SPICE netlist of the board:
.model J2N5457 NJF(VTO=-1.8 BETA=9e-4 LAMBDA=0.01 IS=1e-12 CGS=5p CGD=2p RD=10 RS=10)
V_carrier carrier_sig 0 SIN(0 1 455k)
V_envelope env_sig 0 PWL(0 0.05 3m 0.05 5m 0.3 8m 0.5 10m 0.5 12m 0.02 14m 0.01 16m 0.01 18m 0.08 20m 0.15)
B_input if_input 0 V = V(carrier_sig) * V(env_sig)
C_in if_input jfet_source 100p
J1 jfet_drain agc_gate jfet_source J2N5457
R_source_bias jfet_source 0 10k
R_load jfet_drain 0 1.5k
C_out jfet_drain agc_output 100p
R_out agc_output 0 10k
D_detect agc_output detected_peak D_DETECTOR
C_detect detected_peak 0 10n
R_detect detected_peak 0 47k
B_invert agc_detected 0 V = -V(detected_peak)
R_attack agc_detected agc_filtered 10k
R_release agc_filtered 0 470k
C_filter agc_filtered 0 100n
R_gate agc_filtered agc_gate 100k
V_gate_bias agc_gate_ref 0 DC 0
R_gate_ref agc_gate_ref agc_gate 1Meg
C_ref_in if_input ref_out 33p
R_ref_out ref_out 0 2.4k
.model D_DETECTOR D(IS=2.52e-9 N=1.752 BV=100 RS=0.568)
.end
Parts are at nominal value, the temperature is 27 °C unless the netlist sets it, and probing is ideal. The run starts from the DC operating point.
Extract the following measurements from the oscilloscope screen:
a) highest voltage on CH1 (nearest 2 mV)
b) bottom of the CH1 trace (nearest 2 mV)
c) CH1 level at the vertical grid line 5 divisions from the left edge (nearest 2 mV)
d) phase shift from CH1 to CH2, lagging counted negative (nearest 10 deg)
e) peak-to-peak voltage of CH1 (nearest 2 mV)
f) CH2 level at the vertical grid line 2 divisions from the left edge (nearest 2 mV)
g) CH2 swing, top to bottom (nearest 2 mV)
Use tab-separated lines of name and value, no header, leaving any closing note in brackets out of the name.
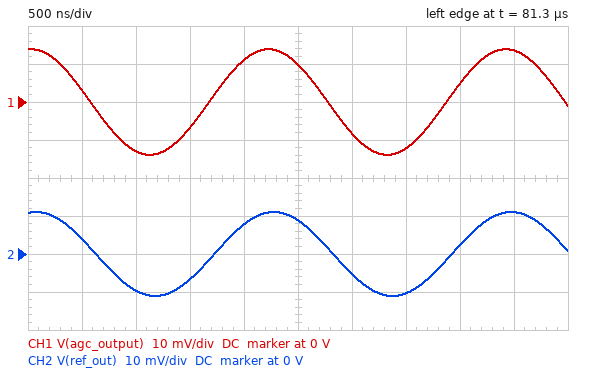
highest voltage on CH1	14 mV
bottom of the CH1 trace	-14 mV
CH1 level at the vertical grid line 5 divisions from the left edge	10 mV
phase shift from CH1 to CH2, lagging counted negative	-10 deg
peak-to-peak voltage of CH1	28 mV
CH2 level at the vertical grid line 2 divisions from the left edge	-10 mV
CH2 swing, top to bottom	22 mV
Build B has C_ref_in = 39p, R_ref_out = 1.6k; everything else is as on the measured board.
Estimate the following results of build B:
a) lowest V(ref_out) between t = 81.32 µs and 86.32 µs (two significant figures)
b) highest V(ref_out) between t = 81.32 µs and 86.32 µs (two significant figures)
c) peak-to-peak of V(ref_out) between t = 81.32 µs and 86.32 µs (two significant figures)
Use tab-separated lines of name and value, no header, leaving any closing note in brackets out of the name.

lowest V(ref_out) between t = 81.32 µs and 86.32 µs	-8.8 mV
highest V(ref_out) between t = 81.32 µs and 86.32 µs	8.8 mV
peak-to-peak of V(ref_out) between t = 81.32 µs and 86.32 µs	18 mV
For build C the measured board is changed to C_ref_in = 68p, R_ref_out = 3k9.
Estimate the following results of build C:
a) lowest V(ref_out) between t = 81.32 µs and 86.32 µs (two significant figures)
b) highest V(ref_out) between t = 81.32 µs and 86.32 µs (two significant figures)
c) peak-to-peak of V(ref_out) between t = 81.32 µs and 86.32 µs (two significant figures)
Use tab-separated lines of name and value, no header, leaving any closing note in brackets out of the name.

lowest V(ref_out) between t = 81.32 µs and 86.32 µs	-30 mV
highest V(ref_out) between t = 81.32 µs and 86.32 µs	30 mV
peak-to-peak of V(ref_out) between t = 81.32 µs and 86.32 µs	60 mV
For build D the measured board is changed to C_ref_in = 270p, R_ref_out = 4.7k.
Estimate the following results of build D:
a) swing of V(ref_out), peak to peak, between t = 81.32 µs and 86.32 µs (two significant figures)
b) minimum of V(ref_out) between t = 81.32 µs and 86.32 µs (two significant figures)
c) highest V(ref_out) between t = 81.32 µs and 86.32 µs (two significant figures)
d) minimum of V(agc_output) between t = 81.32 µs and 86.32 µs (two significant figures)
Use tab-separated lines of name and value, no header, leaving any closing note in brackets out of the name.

swing of V(ref_out), peak to peak, between t = 81.32 µs and 86.32 µs	96 mV
minimum of V(ref_out) between t = 81.32 µs and 86.32 µs	-48 mV
highest V(ref_out) between t = 81.32 µs and 86.32 µs	48 mV
minimum of V(agc_output) between t = 81.32 µs and 86.32 µs	-14 mV
